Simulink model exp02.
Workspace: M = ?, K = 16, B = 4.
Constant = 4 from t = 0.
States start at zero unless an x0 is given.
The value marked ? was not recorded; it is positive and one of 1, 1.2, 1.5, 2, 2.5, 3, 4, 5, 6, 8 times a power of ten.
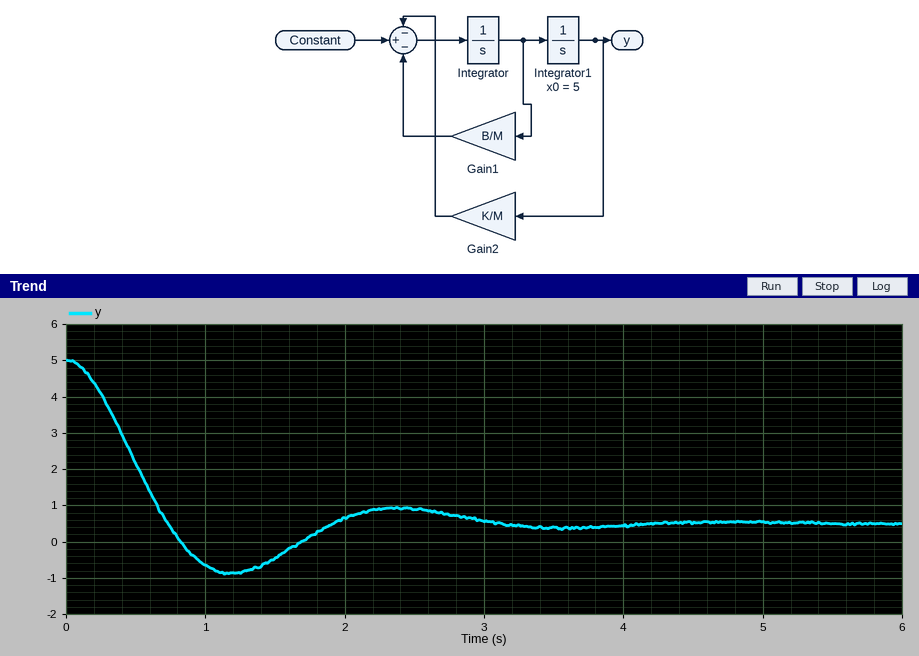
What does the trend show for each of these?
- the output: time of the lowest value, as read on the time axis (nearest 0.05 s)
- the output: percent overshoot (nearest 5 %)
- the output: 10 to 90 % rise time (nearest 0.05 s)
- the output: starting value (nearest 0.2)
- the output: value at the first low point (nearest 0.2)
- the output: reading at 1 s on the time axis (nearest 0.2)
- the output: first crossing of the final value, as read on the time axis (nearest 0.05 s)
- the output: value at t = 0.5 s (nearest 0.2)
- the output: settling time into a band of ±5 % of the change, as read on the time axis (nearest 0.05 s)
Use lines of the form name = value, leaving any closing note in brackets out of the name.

the output: time of the lowest value, as read on the time axis = 1.20 s
the output: percent overshoot = 30 %
the output: 10 to 90 % rise time = 0.50 s
the output: starting value = 5.0
the output: value at the first low point = -0.8
the output: reading at 1 s on the time axis = -0.6
the output: first crossing of the final value, as read on the time axis = 0.75 s
the output: value at t = 0.5 s = 2.2
the output: settling time into a band of ±5 % of the change, as read on the time axis = 2.80 s
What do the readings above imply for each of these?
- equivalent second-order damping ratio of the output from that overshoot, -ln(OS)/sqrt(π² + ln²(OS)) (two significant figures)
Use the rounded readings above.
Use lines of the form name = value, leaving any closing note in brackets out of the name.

equivalent second-order damping ratio of the output from that overshoot, -ln(OS)/sqrt(π² + ln²(OS)) = 0.36
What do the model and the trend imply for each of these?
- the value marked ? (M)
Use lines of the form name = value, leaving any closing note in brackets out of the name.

the value marked ? = 2
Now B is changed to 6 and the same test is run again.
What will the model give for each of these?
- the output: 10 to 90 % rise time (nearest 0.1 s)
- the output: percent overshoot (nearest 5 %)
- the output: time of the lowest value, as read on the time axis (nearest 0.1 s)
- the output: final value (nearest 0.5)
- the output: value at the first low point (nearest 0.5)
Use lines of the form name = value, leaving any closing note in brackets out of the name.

the output: 10 to 90 % rise time = 0.6 s
the output: percent overshoot = 15 %
the output: time of the lowest value, as read on the time axis = 1.3 s
the output: final value = 0.5
the output: value at the first low point = 0.0
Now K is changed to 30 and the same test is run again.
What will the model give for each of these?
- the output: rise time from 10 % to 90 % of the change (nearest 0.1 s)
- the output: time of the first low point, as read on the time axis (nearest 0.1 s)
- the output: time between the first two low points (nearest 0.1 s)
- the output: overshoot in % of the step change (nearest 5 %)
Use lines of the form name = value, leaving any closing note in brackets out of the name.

the output: rise time from 10 % to 90 % of the change = 0.3 s
the output: time of the first low point, as read on the time axis = 0.8 s
the output: time between the first two low points = 1.7 s
the output: overshoot in % of the step change = 45 %
